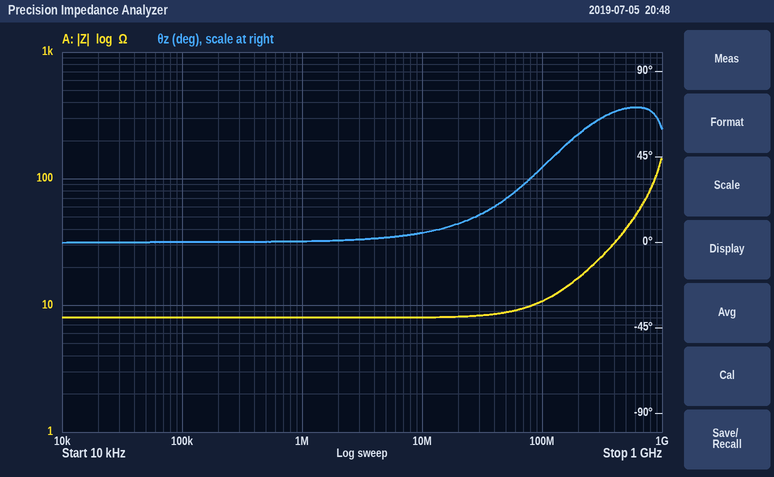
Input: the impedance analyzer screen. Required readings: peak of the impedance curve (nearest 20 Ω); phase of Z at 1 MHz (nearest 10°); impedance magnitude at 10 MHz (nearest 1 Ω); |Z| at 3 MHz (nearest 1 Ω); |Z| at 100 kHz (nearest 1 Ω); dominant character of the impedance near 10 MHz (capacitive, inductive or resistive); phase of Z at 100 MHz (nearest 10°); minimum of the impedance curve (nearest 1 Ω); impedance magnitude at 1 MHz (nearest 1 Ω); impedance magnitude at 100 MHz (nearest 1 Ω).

140 Ω
0°
8 Ω
8 Ω
8 Ω
resistive
40°
8 Ω
8 Ω
11 Ω
